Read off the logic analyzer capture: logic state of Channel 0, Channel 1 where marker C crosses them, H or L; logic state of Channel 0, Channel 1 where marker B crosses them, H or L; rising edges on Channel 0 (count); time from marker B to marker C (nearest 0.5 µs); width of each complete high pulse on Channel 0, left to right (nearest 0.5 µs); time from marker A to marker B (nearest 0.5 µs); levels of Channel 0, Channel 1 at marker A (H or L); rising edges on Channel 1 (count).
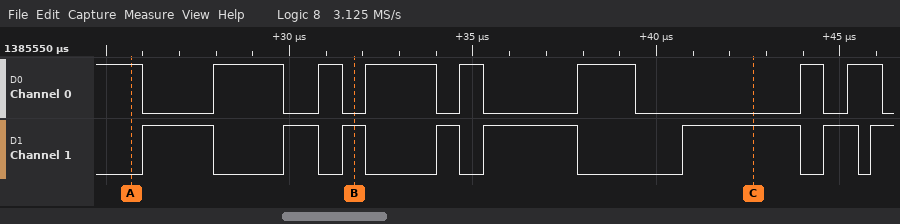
Channel 0=L, Channel 1=H
Channel 0=L, Channel 1=H
7
11 µs
2 µs, 0.5 µs, 2 µs, 0.5 µs, 1.5 µs, 0.5 µs, 1 µs
6 µs
Channel 0=H, Channel 1=L
8
